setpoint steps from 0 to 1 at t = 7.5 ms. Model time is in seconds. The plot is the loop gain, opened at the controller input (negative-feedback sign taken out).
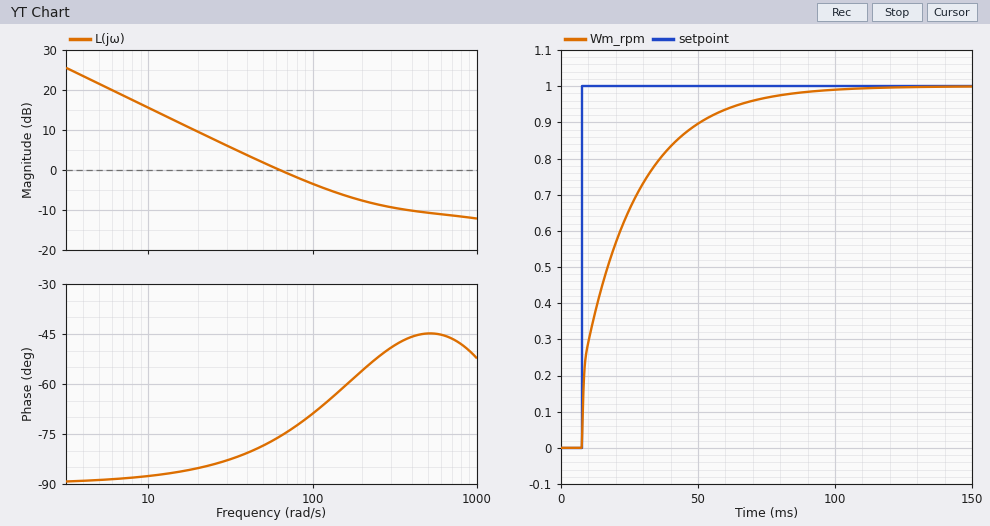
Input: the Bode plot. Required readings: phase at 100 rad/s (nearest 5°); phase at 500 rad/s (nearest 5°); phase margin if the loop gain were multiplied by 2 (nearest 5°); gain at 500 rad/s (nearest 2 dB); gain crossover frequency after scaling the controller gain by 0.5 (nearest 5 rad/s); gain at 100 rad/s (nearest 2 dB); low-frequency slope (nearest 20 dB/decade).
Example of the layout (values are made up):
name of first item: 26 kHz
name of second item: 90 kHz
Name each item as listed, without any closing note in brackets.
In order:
phase at 100 rad/s: -70°
phase at 500 rad/s: -45°
phase margin if the loop gain were multiplied by 2: 120°
gain at 500 rad/s: -10 dB
gain crossover frequency after scaling the controller gain by 0.5: 30 rad/s
gain at 100 rad/s: -4 dB
low-frequency slope: -20 dB/decade
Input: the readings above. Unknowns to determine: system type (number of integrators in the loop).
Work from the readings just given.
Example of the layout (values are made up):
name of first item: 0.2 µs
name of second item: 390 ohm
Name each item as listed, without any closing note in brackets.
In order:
system type: 1
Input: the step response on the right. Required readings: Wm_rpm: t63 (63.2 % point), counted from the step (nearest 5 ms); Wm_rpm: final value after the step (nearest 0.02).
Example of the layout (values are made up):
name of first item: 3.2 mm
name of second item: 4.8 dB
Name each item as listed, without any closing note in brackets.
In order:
Wm_rpm: t63 (63.2 % point), counted from the step: 15 ms
Wm_rpm: final value after the step: 1.00
